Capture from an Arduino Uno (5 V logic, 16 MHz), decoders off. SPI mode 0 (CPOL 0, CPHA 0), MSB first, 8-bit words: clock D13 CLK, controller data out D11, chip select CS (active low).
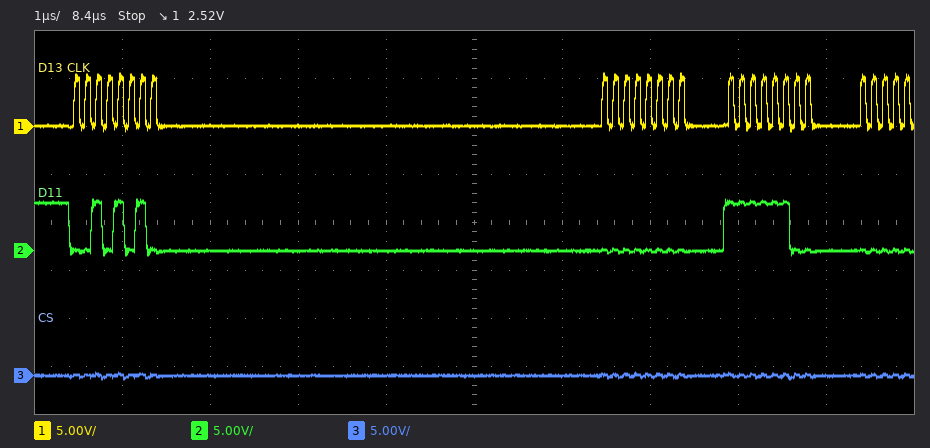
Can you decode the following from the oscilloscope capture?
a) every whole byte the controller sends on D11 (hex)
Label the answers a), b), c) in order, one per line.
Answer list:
a) 2A 00 FC
